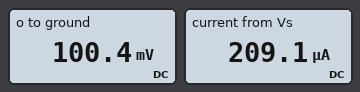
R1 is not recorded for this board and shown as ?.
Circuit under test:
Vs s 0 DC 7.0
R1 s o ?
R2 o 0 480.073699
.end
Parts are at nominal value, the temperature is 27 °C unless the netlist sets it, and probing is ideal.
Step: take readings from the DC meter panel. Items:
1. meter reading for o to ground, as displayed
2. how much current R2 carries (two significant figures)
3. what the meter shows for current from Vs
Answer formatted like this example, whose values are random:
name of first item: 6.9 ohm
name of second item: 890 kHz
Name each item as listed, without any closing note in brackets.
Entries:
meter reading for o to ground, as displayed: 100.4 mV
how much current R2 carries: 210 µA
what the meter shows for current from Vs: 209.1 µA
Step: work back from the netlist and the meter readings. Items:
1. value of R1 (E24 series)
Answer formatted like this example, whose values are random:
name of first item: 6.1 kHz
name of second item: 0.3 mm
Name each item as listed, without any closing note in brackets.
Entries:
value of R1: 33 kΩ
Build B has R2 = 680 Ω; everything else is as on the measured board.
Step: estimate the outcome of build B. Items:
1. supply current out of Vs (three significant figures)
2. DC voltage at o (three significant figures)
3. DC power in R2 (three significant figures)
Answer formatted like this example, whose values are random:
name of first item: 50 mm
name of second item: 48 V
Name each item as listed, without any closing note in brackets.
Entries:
supply current out of Vs: 208 µA
DC voltage at o: 141 mV
DC power in R2: 29.4 µW
